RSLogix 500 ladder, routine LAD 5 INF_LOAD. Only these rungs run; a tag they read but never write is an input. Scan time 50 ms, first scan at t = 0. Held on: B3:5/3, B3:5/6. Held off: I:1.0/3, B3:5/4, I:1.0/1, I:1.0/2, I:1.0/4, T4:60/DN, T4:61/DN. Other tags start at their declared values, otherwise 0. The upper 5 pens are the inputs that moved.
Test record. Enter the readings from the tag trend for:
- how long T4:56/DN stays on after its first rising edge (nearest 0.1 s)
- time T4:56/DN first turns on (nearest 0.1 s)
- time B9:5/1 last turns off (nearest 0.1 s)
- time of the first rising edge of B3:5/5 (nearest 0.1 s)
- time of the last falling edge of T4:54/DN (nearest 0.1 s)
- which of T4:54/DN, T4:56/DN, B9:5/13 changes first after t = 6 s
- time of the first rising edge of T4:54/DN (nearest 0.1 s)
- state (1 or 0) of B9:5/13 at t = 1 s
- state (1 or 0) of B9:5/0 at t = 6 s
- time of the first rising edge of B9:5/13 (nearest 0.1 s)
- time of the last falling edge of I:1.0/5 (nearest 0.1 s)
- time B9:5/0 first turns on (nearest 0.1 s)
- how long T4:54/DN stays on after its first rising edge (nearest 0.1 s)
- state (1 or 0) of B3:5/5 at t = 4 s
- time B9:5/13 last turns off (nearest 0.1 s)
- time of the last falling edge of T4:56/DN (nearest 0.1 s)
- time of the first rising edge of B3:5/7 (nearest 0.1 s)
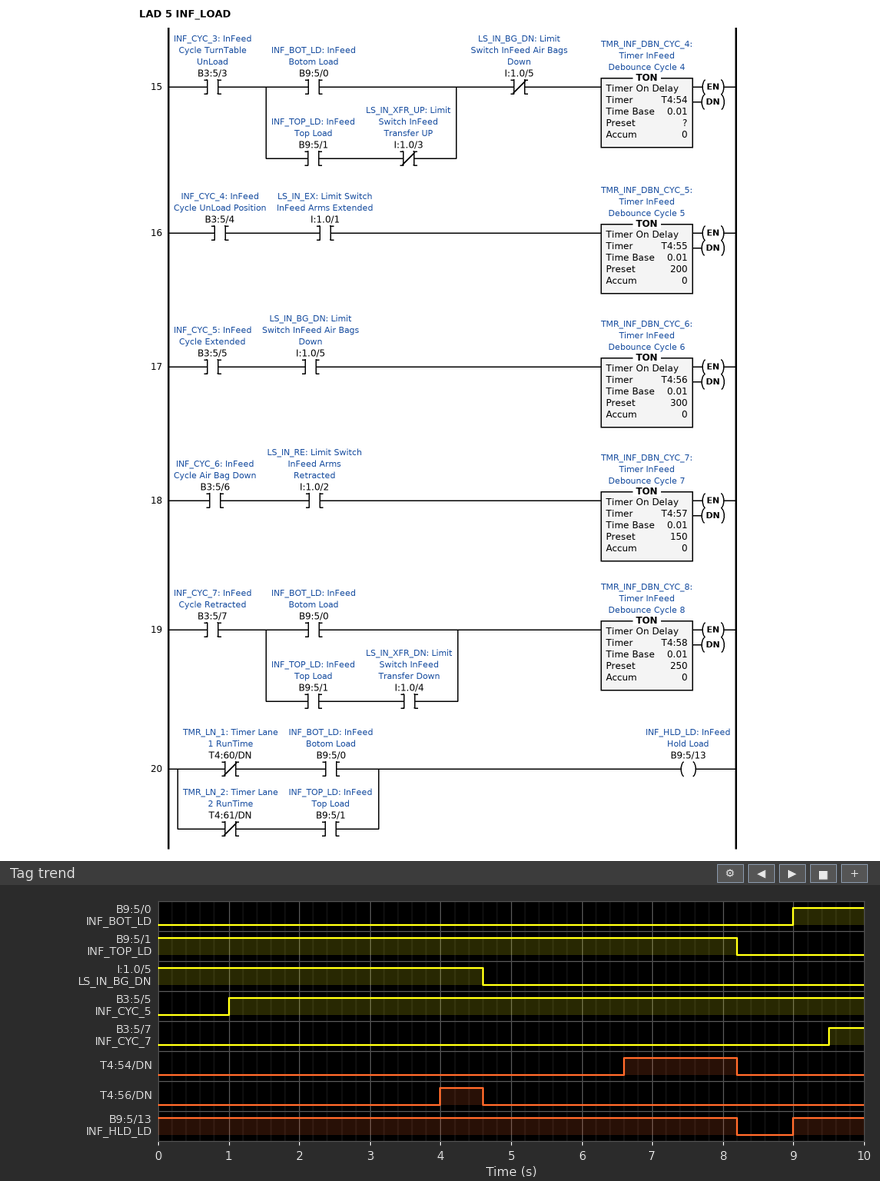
0.6 s
4.0 s
8.2 s
1.0 s
8.2 s
T4:54/DN
6.6 s
1
0
9.0 s
4.6 s
9.0 s
1.6 s
1
8.2 s
4.6 s
9.5 s
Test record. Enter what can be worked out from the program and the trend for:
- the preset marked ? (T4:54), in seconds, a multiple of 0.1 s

2.0 s
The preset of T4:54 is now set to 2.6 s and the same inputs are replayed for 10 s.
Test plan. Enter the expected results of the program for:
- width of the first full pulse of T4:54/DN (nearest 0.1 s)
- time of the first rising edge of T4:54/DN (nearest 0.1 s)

1.0 s
7.2 s
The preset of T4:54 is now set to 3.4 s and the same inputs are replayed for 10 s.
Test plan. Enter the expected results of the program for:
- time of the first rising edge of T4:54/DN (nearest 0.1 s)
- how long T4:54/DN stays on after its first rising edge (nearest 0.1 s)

8.0 s
0.2 s
